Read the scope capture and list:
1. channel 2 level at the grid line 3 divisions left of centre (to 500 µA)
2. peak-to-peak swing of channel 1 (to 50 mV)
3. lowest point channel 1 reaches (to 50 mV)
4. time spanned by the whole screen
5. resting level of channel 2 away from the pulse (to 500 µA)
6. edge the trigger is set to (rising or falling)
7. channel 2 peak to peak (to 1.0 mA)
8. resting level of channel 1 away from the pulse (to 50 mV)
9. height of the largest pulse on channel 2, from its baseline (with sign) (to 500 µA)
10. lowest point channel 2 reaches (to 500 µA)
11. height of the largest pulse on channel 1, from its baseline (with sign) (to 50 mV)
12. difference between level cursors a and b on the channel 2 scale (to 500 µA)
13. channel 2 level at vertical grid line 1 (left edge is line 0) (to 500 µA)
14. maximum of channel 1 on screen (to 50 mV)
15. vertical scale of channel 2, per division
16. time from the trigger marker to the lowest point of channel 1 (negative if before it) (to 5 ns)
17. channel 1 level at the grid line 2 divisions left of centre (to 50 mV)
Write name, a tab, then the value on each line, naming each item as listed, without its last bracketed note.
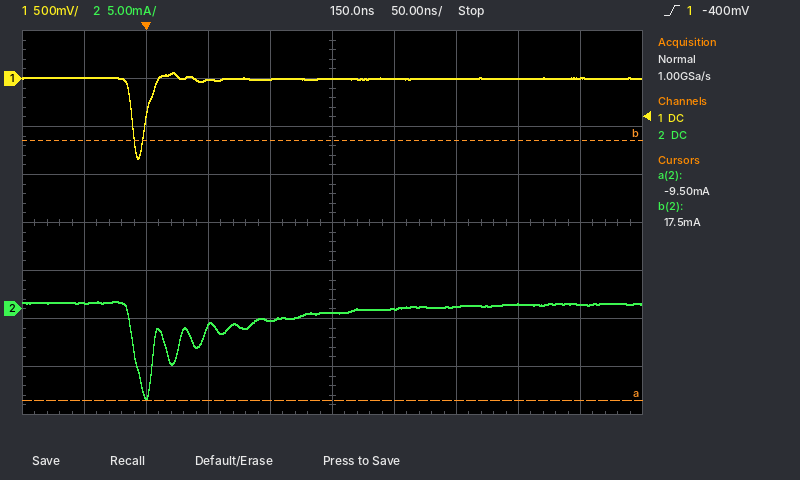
channel 2 level at the grid line 3 divisions left of centre	-9.0 mA
peak-to-peak swing of channel 1	900 mV
lowest point channel 1 reaches	-850 mV
time spanned by the whole screen	500 ns
resting level of channel 2 away from the pulse	500 µA
edge the trigger is set to	rising
channel 2 peak to peak	10.0 mA
resting level of channel 1 away from the pulse	0 mV
height of the largest pulse on channel 2, from its baseline (with sign)	-10.0 mA
lowest point channel 2 reaches	-9.5 mA
height of the largest pulse on channel 1, from its baseline (with sign)	-850 mV
difference between level cursors a and b on the channel 2 scale	27.0 mA
channel 2 level at vertical grid line 1 (left edge is line 0)	500 µA
maximum of channel 1 on screen	50 mV
vertical scale of channel 2, per division	5 mA
time from the trigger marker to the lowest point of channel 1 (negative if before it)	-5 ns
channel 1 level at the grid line 2 divisions left of centre	0 mV
